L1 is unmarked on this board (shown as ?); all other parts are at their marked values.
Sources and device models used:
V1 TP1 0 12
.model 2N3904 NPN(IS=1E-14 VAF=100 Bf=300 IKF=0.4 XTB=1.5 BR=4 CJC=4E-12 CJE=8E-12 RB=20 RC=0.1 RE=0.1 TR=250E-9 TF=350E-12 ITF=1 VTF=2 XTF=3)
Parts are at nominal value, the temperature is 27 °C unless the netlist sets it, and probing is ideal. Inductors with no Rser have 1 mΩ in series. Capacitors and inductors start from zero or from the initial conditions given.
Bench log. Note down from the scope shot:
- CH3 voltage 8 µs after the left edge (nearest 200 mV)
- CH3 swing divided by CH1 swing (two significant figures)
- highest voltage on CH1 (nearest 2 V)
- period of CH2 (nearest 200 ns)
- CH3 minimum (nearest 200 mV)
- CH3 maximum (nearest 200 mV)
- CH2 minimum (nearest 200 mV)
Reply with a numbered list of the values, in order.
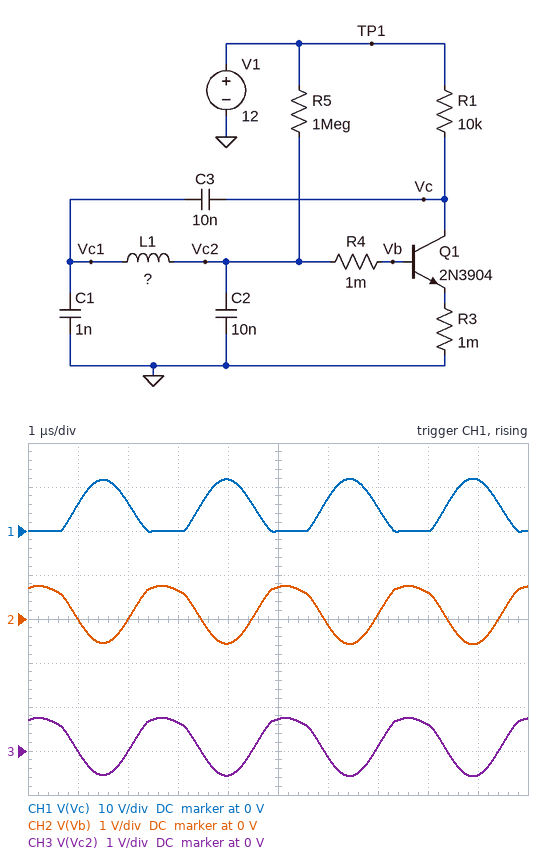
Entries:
1. 600 mV
2. 0.11
3. 12 V
4. 2.4 µs
5. -600 mV
6. 800 mV
7. -600 mV
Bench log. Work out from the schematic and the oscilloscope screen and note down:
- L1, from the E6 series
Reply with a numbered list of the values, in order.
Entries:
1. 150 µH
